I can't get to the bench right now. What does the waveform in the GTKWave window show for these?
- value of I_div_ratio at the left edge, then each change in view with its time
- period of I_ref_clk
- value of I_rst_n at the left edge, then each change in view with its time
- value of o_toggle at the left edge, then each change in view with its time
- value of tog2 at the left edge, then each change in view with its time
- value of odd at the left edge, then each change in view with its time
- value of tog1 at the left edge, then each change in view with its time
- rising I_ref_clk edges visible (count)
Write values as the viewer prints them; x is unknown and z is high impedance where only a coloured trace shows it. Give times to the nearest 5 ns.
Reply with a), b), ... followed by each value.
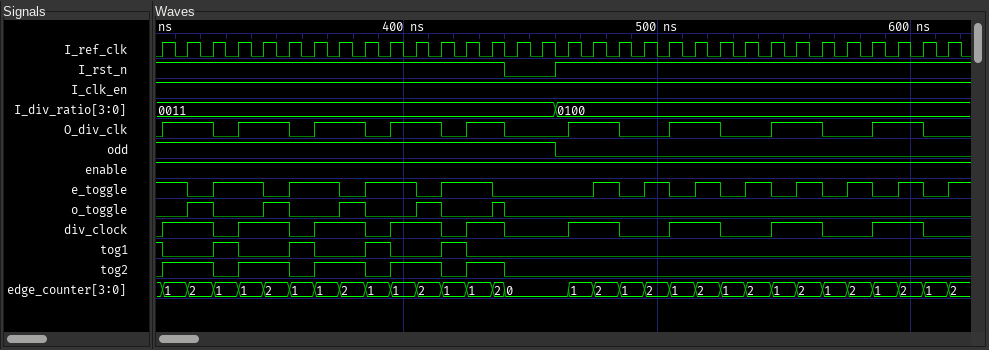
a) 0011, 0100 at 460 ns
b) 10 ns
c) 1, 0 at 440 ns, 1 at 460 ns
d) 0, 1 at 315 ns, 0 at 325 ns, 1 at 345 ns, 0 at 355 ns, 1 at 375 ns, 0 at 385 ns, 1 at 405 ns, 0 at 415 ns, 1 at 435 ns, 0 at 440 ns
e) 0, 1 at 305 ns, 0 at 325 ns, 1 at 335 ns, 0 at 355 ns, 1 at 365 ns, 0 at 385 ns, 1 at 395 ns, 0 at 415 ns, 1 at 425 ns, 0 at 440 ns
f) 1, 0 at 460 ns
g) 1, 0 at 305 ns, 1 at 325 ns, 0 at 335 ns, 1 at 355 ns, 0 at 365 ns, 1 at 385 ns, 0 at 395 ns, 1 at 415 ns, 0 at 425 ns
h) 32
